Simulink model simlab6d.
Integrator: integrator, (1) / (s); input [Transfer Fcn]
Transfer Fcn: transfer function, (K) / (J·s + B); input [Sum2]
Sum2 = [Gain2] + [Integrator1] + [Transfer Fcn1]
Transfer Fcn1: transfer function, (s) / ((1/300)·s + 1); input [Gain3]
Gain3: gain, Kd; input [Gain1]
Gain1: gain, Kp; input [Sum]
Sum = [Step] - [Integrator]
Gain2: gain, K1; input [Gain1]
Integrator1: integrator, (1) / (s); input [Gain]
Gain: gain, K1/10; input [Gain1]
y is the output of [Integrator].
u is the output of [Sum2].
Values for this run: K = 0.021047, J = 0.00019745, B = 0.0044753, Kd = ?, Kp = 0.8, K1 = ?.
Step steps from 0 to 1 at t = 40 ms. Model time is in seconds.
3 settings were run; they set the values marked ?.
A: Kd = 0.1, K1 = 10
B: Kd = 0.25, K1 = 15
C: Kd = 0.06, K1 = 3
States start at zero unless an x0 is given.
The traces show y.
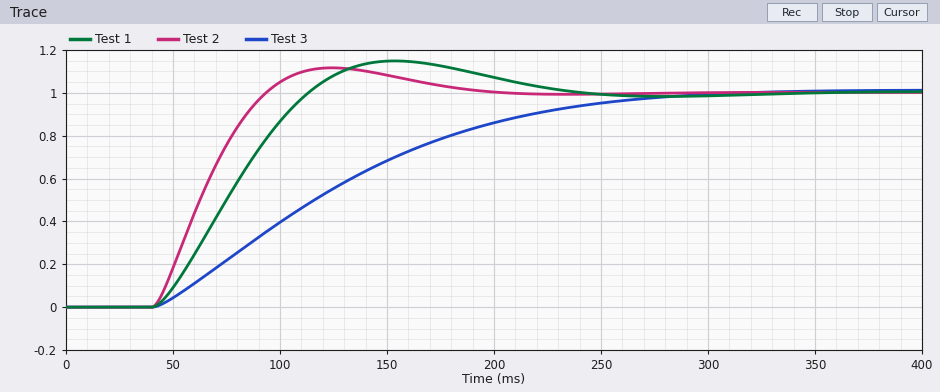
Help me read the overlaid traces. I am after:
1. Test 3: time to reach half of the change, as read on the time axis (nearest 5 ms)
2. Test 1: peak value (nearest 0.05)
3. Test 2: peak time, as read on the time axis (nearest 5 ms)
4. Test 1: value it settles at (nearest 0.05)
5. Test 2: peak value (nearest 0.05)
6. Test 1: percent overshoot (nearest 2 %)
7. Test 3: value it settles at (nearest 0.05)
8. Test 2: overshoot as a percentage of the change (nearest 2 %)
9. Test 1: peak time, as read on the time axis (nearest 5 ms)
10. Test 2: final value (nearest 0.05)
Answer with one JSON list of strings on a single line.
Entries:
["115 ms", "1.15", "125 ms", "1.00", "1.10", "14 %", "1.00", "12 %", "155 ms", "1.00"]
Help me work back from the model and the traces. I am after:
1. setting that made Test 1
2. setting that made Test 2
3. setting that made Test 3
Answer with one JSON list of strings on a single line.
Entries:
["A", "B", "C"]
